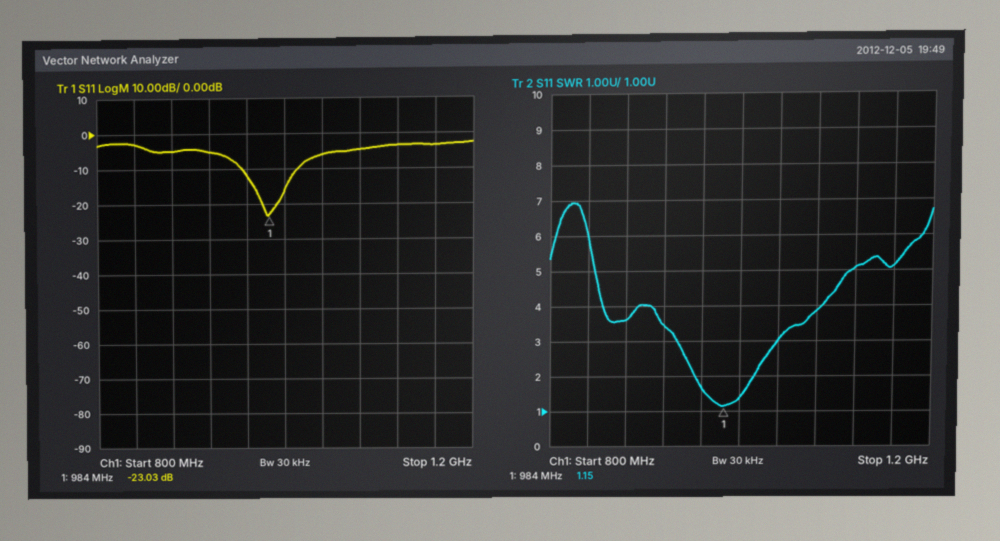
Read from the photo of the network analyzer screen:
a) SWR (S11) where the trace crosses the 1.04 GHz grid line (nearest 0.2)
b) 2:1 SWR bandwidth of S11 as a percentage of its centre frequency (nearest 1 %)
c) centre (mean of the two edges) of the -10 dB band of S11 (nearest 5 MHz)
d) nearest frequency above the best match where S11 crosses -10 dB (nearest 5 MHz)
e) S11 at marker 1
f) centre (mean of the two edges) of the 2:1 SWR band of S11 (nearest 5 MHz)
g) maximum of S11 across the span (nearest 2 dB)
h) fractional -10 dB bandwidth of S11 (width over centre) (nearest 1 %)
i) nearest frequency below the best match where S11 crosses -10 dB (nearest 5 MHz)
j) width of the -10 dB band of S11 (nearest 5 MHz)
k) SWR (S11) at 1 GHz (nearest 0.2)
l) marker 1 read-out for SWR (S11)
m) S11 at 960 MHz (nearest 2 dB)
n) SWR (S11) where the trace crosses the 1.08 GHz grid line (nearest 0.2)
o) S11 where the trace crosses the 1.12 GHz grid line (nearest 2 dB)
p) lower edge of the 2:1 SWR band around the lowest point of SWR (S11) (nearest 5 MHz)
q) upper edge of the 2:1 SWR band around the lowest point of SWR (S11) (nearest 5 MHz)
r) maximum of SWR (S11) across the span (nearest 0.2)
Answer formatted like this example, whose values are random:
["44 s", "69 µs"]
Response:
["3.0", "6 %", "985 MHz", "1.015 GHz", "-23.03 dB", "985 MHz", "-2 dB", "6 %", "955 MHz", "60 MHz", "1.4", "1.15", "-12 dB", "3.8", "-4 dB", "955 MHz", "1.015 GHz", "7.0"]
